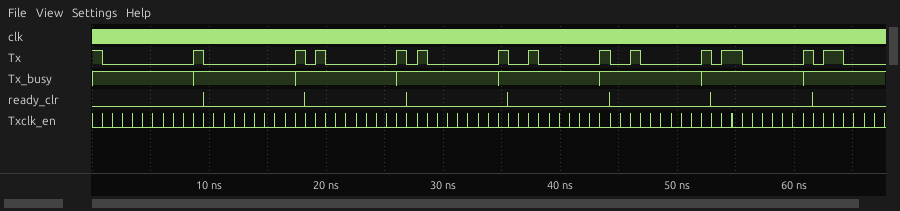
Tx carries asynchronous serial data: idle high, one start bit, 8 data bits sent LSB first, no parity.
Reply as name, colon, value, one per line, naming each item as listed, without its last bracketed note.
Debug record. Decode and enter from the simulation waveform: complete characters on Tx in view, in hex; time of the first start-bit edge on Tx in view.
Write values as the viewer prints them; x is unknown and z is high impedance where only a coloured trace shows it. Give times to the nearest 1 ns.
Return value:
complete characters on Tx in view, in hex: 00, 00, 01, 01, 02, 02, 03
time of the first start-bit edge on Tx in view: 1 ns
